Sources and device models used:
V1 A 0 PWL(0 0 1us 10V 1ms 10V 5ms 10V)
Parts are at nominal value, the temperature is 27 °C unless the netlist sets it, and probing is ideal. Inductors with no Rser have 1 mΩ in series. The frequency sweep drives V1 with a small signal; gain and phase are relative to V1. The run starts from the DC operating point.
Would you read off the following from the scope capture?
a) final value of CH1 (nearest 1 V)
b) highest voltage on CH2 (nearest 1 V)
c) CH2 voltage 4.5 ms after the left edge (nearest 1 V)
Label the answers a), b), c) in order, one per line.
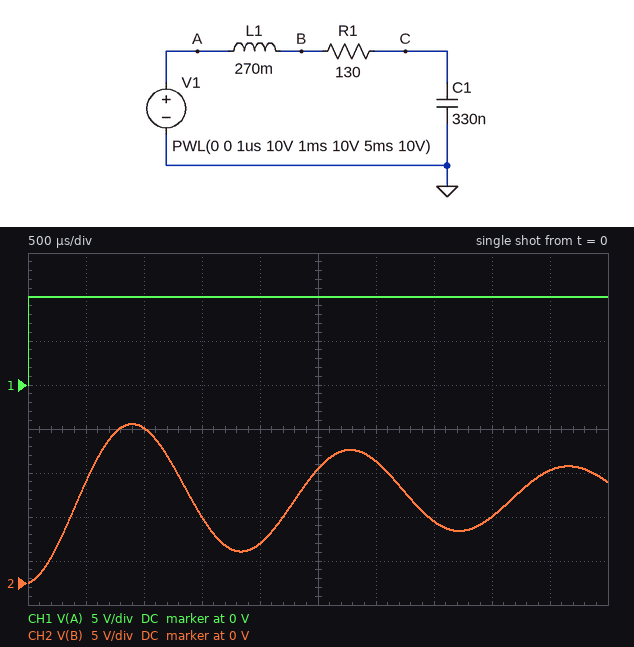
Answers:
a) 10 V
b) 18 V
c) 13 V
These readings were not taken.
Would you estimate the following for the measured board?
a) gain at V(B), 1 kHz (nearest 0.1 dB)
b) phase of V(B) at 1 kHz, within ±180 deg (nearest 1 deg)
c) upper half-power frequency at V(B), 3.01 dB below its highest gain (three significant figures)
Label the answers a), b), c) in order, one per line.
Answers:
a) -7.8 dB
b) -159 deg
c) 568 Hz
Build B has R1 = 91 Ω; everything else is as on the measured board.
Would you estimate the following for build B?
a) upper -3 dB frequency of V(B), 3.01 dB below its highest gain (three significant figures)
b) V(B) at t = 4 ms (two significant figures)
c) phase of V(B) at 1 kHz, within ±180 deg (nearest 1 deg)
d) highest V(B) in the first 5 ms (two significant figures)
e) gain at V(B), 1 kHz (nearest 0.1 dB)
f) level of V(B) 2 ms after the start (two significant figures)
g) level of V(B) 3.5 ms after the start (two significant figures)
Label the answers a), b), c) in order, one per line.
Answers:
a) 558 Hz
b) 6.7 V
c) -165 deg
d) 19 V
e) -7.9 dB
f) 3.6 V
g) 6.2 V
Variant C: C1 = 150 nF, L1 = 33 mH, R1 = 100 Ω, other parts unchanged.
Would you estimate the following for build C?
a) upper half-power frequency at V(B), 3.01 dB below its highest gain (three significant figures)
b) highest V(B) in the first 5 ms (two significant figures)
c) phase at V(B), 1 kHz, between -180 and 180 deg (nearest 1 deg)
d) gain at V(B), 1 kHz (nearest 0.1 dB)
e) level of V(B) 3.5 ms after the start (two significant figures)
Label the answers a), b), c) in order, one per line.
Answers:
a) 2.47 kHz
b) 17 V
c) -1 deg
d) 1.9 dB
e) 10 V
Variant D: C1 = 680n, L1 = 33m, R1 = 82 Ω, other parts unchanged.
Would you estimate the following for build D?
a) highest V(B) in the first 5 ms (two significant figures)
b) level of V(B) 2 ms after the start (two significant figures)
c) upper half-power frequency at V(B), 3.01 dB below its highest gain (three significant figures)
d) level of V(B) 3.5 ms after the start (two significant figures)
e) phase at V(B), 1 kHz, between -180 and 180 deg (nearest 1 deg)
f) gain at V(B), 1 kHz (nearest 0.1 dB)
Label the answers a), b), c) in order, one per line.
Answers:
a) 16 V
b) 9.4 V
c) 1.22 kHz
d) 10 V
e) -53 deg
f) 9.2 dB
